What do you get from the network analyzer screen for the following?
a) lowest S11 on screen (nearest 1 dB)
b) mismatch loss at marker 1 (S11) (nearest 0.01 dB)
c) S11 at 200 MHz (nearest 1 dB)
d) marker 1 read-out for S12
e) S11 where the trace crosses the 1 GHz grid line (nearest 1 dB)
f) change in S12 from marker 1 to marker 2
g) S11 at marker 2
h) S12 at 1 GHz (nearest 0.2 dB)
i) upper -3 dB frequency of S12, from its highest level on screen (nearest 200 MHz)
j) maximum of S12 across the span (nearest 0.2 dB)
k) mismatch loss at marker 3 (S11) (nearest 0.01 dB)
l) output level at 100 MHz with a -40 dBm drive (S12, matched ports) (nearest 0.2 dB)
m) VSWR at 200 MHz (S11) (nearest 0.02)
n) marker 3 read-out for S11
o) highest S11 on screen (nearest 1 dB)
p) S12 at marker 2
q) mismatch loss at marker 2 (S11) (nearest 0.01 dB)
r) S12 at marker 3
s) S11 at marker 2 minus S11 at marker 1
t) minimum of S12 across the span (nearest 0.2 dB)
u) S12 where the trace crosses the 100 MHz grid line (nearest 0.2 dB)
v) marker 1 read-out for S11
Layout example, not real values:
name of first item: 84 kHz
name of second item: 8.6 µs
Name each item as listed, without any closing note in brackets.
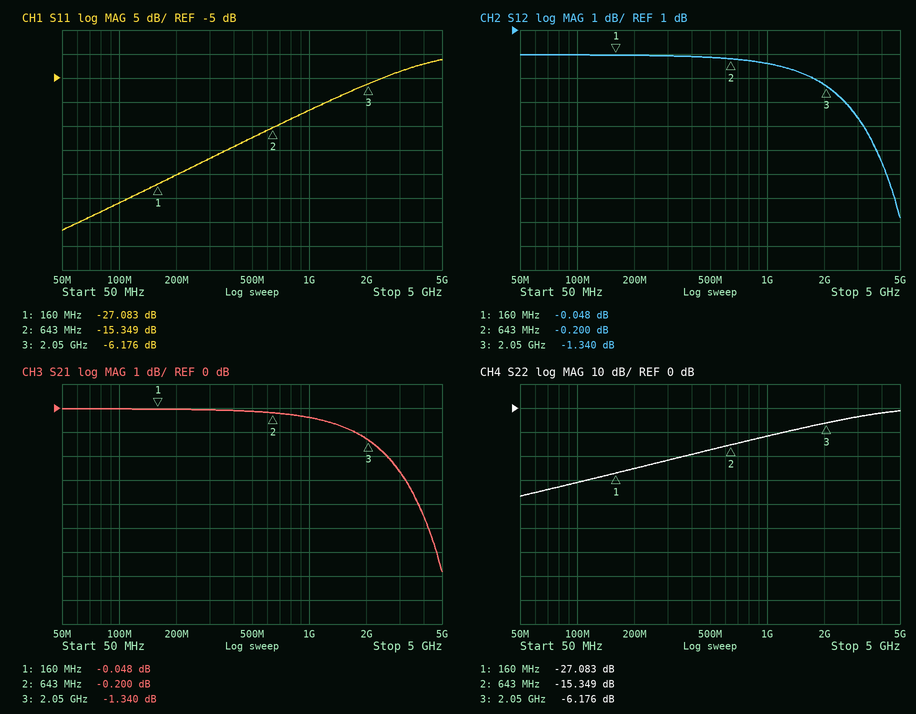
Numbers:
lowest S11 on screen: -37 dB
mismatch loss at marker 1 (S11): 0.01 dB
S11 at 200 MHz: -25 dB
marker 1 read-out for S12: -0.048 dB
S11 where the trace crosses the 1 GHz grid line: -12 dB
change in S12 from marker 1 to marker 2: -0.152 dB
S11 at marker 2: -15.349 dB
S12 at 1 GHz: -0.4 dB
upper -3 dB frequency of S12, from its highest level on screen: 3.2 GHz
maximum of S12 across the span: 0.0 dB
mismatch loss at marker 3 (S11): 1.20 dB
output level at 100 MHz with a -40 dBm drive (S12, matched ports): -40.0 dBm
VSWR at 200 MHz (S11): 1.12
marker 3 read-out for S11: -6.176 dB
highest S11 on screen: -1 dB
S12 at marker 2: -0.200 dB
mismatch loss at marker 2 (S11): 0.13 dB
S12 at marker 3: -1.340 dB
S11 at marker 2 minus S11 at marker 1: 11.734 dB
minimum of S12 across the span: -6.8 dB
S12 where the trace crosses the 100 MHz grid line: 0.0 dB
marker 1 read-out for S11: -27.083 dB
